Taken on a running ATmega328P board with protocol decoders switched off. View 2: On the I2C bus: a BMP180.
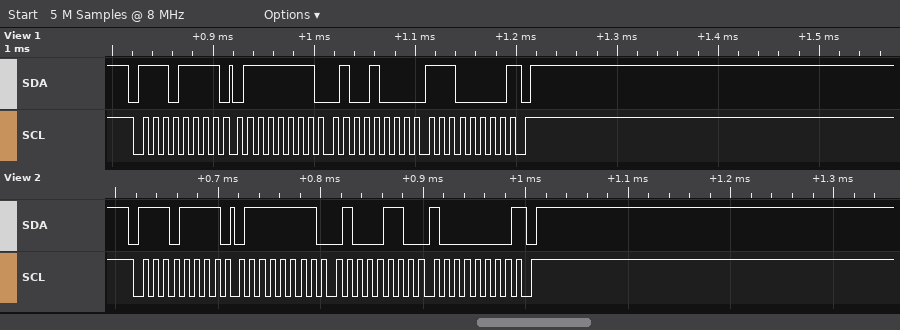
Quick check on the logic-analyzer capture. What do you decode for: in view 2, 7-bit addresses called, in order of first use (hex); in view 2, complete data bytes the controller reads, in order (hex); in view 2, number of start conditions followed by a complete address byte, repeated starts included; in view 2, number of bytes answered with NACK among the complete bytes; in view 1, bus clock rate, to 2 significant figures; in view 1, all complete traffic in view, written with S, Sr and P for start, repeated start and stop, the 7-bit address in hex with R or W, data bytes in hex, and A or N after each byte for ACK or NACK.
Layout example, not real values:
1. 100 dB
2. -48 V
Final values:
1. 0x77
2. 7F 46 80
3. 1
4. 1
5. 100 kHz
6. S 77R A 7F A 48 A E0 N P
